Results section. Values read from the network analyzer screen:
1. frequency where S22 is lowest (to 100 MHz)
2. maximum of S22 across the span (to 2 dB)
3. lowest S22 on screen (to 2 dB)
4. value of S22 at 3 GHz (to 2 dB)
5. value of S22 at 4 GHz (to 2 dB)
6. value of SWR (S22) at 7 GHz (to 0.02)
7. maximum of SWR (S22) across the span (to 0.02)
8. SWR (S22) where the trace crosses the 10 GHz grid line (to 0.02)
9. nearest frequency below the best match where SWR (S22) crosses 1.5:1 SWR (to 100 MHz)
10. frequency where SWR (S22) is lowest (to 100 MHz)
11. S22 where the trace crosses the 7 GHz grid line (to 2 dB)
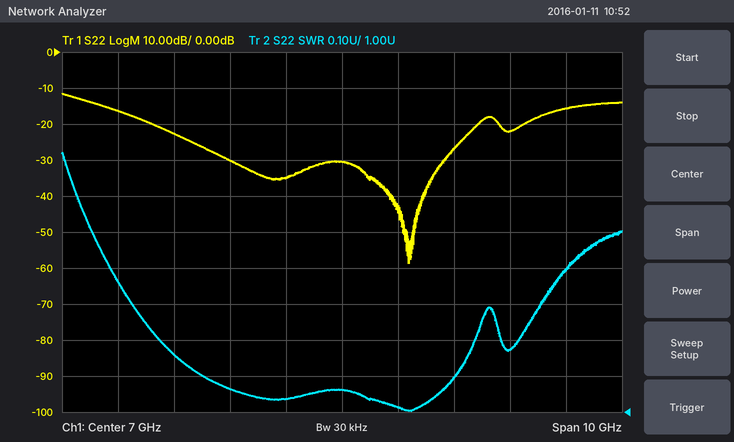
8.2 GHz
-12 dB
-58 dB
-16 dB
-22 dB
1.06
1.72
1.18
2.5 GHz
8.2 GHz
-30 dB
